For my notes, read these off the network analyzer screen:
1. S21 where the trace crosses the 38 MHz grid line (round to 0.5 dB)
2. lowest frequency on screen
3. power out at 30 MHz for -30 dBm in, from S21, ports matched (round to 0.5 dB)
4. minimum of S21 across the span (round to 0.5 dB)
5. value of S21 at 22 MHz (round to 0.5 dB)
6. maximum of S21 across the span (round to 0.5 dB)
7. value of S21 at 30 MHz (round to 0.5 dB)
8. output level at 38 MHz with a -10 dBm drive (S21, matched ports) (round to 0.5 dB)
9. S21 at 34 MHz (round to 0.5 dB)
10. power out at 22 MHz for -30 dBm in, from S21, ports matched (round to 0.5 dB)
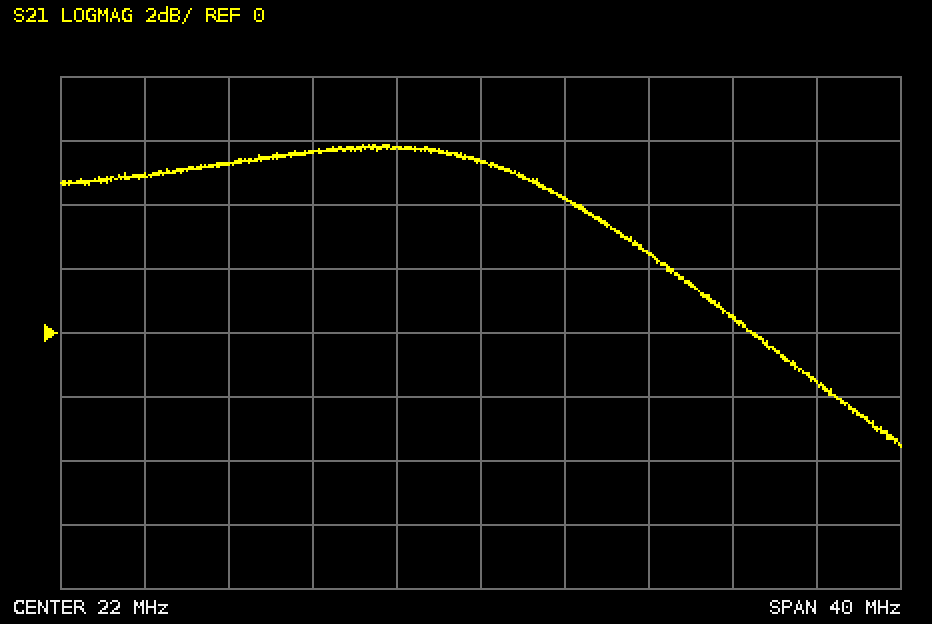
-1.5 dB
2 MHz
-27.5 dBm
-3.5 dB
5.5 dB
6.0 dB
2.5 dB
-11.5 dBm
0.5 dB
-24.5 dBm
